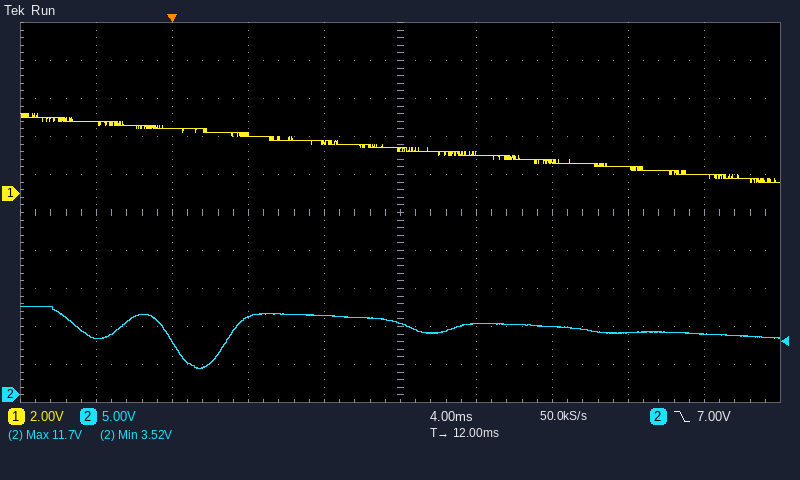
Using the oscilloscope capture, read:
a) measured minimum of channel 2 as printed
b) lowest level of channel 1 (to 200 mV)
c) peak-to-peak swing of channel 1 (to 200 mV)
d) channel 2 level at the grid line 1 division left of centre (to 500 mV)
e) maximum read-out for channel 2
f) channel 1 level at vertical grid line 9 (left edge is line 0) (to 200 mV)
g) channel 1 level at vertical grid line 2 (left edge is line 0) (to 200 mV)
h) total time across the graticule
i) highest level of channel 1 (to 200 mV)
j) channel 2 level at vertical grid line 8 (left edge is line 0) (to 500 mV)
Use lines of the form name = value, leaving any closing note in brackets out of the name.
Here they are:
measured minimum of channel 2 as printed = 3.52 V
lowest level of channel 1 = 600 mV
peak-to-peak swing of channel 1 = 3.6 V
channel 2 level at the grid line 1 division left of centre = 10.5 V
maximum read-out for channel 2 = 11.7 V
channel 1 level at vertical grid line 9 (left edge is line 0) = 1.0 V
channel 1 level at vertical grid line 2 (left edge is line 0) = 3.4 V
total time across the graticule = 40 ms
highest level of channel 1 = 4.2 V
channel 2 level at vertical grid line 8 (left edge is line 0) = 8.0 V
